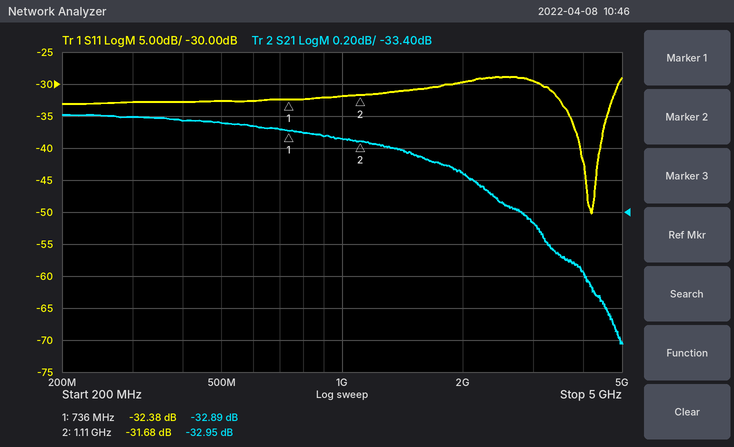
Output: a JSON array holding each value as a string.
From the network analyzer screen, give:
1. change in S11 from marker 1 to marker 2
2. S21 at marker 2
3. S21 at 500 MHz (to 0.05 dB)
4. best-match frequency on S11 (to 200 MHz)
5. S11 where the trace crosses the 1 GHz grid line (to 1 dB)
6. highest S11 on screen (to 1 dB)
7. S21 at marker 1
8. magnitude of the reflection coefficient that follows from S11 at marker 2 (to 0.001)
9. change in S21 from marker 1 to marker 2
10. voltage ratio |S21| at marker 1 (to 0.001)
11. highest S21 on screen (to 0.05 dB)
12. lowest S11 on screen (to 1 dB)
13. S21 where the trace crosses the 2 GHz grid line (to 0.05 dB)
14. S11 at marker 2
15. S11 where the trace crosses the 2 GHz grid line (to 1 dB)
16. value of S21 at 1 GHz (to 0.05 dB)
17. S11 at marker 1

["0.70 dB", "-32.95 dB", "-32.85 dB", "4.2 GHz", "-32 dB", "-29 dB", "-32.89 dB", "0.026", "-0.06 dB", "0.023", "-32.80 dB", "-50 dB", "-33.15 dB", "-31.68 dB", "-30 dB", "-32.95 dB", "-32.38 dB"]
